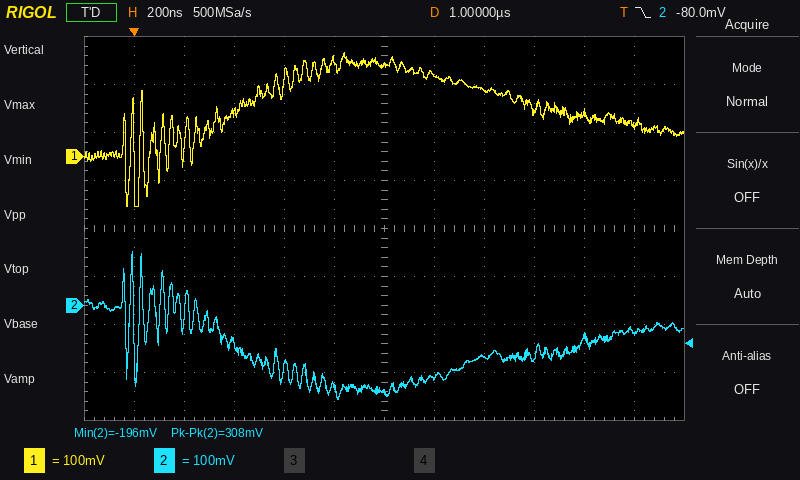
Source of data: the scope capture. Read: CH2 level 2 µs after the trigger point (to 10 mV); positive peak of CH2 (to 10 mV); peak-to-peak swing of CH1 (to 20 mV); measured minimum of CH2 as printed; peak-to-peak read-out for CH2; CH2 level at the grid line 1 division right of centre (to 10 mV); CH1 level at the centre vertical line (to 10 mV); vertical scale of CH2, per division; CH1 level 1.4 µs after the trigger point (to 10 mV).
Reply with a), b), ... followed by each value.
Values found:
a) -60 mV
b) 110 mV
c) 320 mV
d) -196 mV
e) 308 mV
f) -150 mV
g) 190 mV
h) 100 mV
i) 140 mV
